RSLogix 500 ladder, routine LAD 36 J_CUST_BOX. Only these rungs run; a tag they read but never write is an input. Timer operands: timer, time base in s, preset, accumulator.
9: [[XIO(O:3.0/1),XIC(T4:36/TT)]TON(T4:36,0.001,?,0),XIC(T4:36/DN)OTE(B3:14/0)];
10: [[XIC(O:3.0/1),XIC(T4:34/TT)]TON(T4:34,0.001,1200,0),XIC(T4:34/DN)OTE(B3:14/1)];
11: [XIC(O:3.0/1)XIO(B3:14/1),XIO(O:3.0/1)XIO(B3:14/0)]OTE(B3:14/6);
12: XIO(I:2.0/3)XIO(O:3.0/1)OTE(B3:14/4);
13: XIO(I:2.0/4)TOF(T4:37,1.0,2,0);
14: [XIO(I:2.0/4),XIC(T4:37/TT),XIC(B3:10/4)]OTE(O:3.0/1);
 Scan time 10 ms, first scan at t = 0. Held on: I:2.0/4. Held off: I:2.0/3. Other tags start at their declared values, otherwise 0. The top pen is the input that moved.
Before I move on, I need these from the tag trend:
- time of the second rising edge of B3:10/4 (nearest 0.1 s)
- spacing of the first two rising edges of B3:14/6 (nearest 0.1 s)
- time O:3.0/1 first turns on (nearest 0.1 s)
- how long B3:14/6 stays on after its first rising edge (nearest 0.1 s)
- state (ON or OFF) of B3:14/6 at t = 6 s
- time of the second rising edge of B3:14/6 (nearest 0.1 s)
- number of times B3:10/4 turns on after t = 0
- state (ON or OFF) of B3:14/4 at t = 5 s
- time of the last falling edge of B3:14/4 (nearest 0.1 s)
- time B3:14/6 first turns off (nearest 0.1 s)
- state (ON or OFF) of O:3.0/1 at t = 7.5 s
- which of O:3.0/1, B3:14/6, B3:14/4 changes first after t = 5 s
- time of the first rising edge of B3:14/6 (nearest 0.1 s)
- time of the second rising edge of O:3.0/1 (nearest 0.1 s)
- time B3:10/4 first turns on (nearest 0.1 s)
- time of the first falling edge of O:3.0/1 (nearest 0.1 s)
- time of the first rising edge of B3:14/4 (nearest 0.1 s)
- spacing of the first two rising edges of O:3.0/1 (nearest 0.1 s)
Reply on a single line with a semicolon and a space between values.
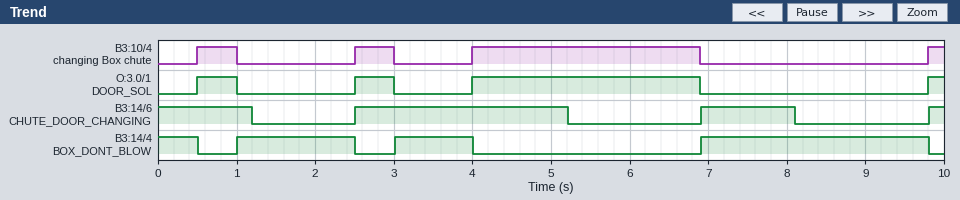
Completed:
2.5 s; 4.4 s; 0.5 s; 2.7 s; OFF; 6.9 s; 4; OFF; 9.8 s; 1.2 s; OFF; B3:14/6; 2.5 s; 2.5 s; 0.5 s; 1.0 s; 1.0 s; 2.0 s
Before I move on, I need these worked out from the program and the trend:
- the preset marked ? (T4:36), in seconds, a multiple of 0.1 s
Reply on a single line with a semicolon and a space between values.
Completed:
1.2 s
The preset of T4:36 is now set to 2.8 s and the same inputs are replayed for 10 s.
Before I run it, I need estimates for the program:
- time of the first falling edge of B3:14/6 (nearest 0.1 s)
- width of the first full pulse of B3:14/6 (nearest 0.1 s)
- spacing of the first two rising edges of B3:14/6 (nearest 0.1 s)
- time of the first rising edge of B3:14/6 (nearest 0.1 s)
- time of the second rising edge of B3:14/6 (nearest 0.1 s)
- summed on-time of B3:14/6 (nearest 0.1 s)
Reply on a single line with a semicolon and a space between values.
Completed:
5.2 s; 2.8 s; 2.9 s; 6.9 s; 9.8 s; 8.2 s
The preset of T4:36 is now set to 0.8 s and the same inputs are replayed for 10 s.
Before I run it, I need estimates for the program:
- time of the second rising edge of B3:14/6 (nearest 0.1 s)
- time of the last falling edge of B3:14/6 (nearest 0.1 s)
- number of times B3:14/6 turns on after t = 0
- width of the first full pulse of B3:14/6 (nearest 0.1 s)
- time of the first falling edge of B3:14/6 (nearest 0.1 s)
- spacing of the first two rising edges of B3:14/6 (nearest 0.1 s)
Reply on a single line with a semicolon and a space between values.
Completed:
4.0 s; 7.7 s; 4; 1.3 s; 1.8 s; 1.5 s
